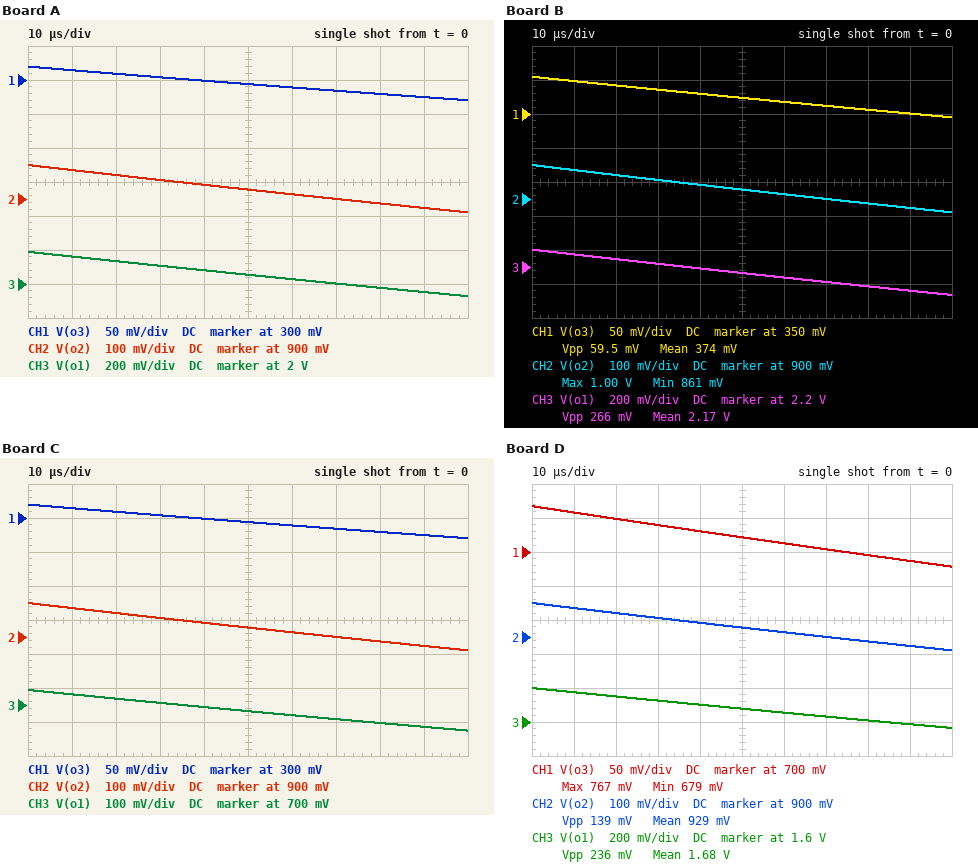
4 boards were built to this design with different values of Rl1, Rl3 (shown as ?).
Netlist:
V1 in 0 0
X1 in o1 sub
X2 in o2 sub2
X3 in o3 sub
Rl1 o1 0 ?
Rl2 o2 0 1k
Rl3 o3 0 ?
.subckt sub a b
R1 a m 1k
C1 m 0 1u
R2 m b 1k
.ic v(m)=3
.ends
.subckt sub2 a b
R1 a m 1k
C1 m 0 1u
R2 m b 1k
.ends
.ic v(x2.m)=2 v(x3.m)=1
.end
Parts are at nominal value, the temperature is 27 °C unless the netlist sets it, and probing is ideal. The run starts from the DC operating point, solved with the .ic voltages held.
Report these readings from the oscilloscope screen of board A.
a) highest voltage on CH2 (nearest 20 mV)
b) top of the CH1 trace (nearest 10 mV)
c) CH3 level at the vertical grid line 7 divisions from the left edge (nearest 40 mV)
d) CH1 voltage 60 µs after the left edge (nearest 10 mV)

1.00 V
320 mV
2.00 V
290 mV
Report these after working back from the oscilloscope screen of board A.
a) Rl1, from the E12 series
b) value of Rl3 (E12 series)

2.7 kΩ
470 Ω
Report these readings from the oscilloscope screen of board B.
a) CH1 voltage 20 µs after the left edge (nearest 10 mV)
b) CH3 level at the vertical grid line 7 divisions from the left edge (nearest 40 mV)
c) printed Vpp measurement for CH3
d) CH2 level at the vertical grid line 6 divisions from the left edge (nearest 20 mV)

390 mV
2.12 V
266 mV
920 mV
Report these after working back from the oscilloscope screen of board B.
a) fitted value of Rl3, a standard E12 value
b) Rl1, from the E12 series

680 Ω
3.3 kΩ
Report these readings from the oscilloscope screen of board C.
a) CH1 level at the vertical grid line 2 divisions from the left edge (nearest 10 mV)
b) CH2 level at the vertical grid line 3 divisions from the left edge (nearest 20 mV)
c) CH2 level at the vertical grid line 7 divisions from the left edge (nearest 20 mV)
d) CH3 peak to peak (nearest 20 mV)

310 mV
960 mV
900 mV
120 mV
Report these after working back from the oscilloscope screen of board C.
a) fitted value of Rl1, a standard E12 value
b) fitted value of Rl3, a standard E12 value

330 Ω
470 Ω
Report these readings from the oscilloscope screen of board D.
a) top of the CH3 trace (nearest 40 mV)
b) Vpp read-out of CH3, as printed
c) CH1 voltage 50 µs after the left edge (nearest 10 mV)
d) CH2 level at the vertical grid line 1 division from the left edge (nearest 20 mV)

1.80 V
236 mV
720 mV
980 mV
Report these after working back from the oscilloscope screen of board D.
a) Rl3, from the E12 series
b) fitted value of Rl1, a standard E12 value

3.3 kΩ
1.5 kΩ
